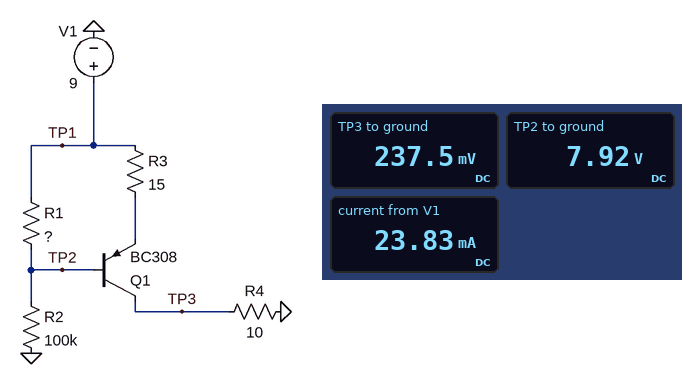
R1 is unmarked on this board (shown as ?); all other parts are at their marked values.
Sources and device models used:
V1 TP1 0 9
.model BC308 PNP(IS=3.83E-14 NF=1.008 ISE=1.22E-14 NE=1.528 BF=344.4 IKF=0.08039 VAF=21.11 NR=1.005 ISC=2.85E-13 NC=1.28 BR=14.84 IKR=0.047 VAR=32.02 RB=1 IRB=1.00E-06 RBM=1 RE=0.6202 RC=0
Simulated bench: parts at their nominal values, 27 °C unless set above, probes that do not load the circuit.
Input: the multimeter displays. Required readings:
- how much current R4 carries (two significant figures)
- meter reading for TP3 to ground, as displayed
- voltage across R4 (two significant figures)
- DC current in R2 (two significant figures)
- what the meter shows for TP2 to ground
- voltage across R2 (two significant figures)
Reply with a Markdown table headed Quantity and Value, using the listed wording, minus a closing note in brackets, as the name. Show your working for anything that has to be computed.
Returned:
| Quantity | Value |
|---|---|
| how much current R4 carries | (237.5 mV) / 10 Ω = 24 mA |
| meter reading for TP3 to ground, as displayed | 237.5 mV |
| voltage across R4 | 237.5 mV = 240 mV |
| DC current in R2 | (7.92 V) / 100 kΩ = 79 µA |
| what the meter shows for TP2 to ground | 7.92 V |
| voltage across R2 | 7.92 V = 7.9 V |
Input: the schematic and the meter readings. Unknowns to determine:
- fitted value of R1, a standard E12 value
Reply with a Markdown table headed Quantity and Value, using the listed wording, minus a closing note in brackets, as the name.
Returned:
| Quantity | Value |
|---|---|
| fitted value of R1, a standard E12 value | 68 kΩ |
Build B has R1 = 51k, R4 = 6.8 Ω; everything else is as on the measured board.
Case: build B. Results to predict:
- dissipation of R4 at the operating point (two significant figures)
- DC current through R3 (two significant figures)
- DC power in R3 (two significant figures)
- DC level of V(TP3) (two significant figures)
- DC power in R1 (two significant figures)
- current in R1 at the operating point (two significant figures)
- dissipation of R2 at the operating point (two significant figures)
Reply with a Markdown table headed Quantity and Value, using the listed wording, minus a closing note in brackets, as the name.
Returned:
| Quantity | Value |
|---|---|
| dissipation of R4 at the operating point | 3.4 mW |
| DC current through R3 | 22 mA |
| DC power in R3 | 7.5 mW |
| DC level of V(TP3) | 150 mV |
| DC power in R1 | 22 µW |
| current in R1 at the operating point | 21 µA |
| dissipation of R2 at the operating point | 630 µW |
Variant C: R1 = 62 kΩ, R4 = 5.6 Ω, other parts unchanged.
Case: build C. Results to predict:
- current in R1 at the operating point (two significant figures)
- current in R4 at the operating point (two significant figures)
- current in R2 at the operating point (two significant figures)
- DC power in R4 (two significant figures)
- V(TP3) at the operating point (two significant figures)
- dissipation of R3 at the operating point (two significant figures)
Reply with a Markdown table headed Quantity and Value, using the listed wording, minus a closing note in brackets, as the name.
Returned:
| Quantity | Value |
|---|---|
| current in R1 at the operating point | 17 µA |
| current in R4 at the operating point | 23 mA |
| current in R2 at the operating point | 79 µA |
| DC power in R4 | 3.1 mW |
| V(TP3) at the operating point | 130 mV |
| dissipation of R3 at the operating point | 8.3 mW |
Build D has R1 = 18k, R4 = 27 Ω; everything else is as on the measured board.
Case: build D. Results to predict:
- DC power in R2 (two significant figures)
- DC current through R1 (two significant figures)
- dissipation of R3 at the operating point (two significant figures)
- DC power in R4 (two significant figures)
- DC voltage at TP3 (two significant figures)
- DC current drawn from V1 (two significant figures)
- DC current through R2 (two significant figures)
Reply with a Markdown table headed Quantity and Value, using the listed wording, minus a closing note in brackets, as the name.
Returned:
| Quantity | Value |
|---|---|
| DC power in R2 | 660 µW |
| DC current through R1 | 49 µA |
| dissipation of R3 at the operating point | 2.5 mW |
| DC power in R4 | 4.5 mW |
| DC voltage at TP3 | 350 mV |
| DC current drawn from V1 | 13 mA |
| DC current through R2 | 81 µA |
